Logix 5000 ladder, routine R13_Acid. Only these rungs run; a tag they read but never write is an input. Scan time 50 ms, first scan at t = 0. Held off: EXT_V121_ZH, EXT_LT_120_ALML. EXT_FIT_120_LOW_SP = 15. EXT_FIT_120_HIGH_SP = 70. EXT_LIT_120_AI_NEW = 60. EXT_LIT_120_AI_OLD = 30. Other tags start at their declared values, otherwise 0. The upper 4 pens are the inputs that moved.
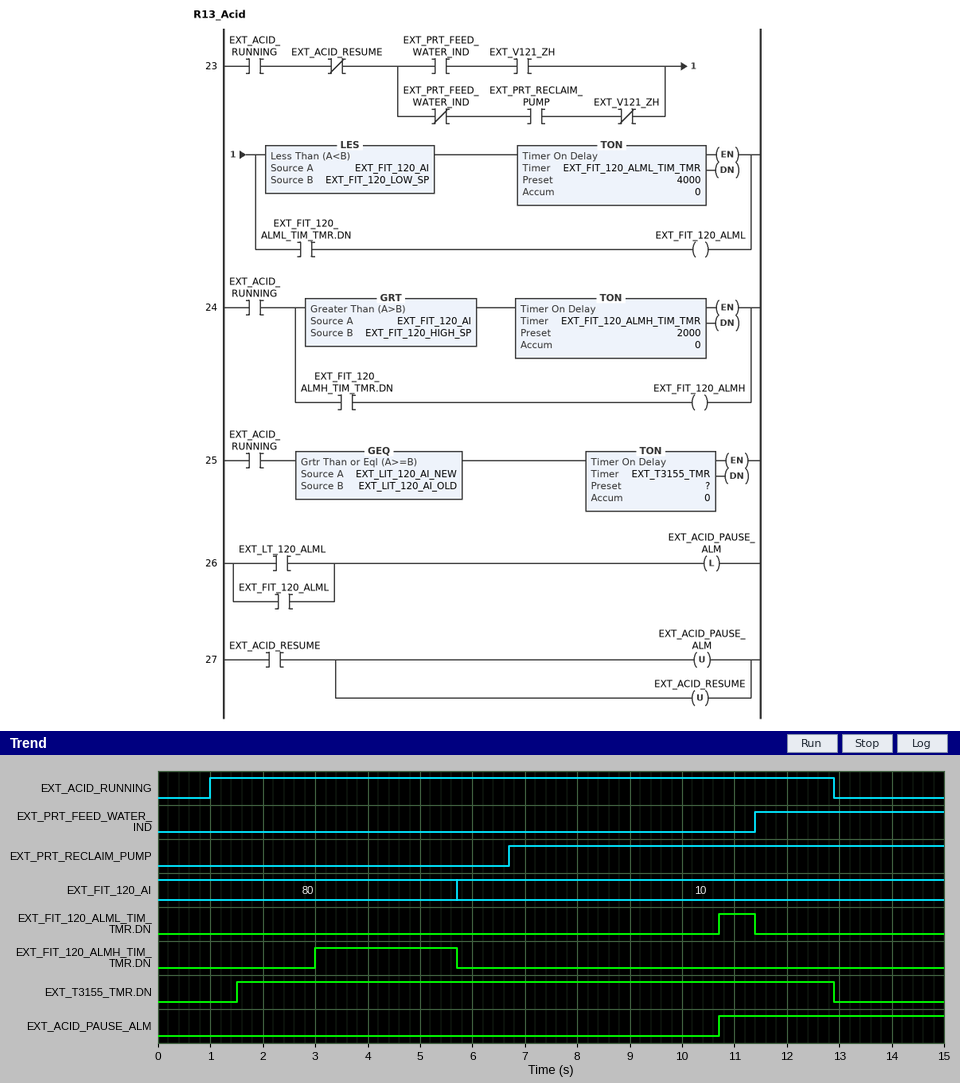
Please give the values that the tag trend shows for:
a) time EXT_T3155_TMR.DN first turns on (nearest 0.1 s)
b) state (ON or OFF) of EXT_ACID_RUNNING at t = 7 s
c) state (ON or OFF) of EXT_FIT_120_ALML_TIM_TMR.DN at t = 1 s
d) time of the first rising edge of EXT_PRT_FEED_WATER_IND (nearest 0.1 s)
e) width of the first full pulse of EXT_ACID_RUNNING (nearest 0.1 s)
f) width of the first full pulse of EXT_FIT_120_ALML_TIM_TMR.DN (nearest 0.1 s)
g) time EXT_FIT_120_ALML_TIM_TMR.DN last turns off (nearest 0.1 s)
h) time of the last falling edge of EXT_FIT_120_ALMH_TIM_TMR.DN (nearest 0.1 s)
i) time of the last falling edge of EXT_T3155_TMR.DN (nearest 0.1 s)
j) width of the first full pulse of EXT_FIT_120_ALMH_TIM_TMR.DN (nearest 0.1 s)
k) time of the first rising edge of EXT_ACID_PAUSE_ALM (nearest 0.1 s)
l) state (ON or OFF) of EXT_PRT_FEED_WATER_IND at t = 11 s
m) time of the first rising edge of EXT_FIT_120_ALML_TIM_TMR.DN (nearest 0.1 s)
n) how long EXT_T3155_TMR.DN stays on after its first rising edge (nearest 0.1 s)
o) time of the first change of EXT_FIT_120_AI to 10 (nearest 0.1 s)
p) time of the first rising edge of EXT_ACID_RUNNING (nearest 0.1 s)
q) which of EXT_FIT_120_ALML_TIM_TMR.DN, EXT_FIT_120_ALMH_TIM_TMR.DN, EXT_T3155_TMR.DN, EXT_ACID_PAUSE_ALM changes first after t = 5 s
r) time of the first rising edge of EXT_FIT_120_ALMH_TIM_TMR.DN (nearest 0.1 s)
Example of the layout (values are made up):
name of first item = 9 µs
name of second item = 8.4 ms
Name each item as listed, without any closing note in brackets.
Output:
time EXT_T3155_TMR.DN first turns on = 1.5 s
state (ON or OFF) of EXT_ACID_RUNNING at t = 7 s = ON
state (ON or OFF) of EXT_FIT_120_ALML_TIM_TMR.DN at t = 1 s = OFF
time of the first rising edge of EXT_PRT_FEED_WATER_IND = 11.4 s
width of the first full pulse of EXT_ACID_RUNNING = 11.9 s
width of the first full pulse of EXT_FIT_120_ALML_TIM_TMR.DN = 0.7 s
time EXT_FIT_120_ALML_TIM_TMR.DN last turns off = 11.4 s
time of the last falling edge of EXT_FIT_120_ALMH_TIM_TMR.DN = 5.7 s
time of the last falling edge of EXT_T3155_TMR.DN = 12.9 s
width of the first full pulse of EXT_FIT_120_ALMH_TIM_TMR.DN = 2.7 s
time of the first rising edge of EXT_ACID_PAUSE_ALM = 10.7 s
state (ON or OFF) of EXT_PRT_FEED_WATER_IND at t = 11 s = OFF
time of the first rising edge of EXT_FIT_120_ALML_TIM_TMR.DN = 10.7 s
how long EXT_T3155_TMR.DN stays on after its first rising edge = 11.4 s
time of the first change of EXT_FIT_120_AI to 10 = 5.7 s
time of the first rising edge of EXT_ACID_RUNNING = 1.0 s
which of EXT_FIT_120_ALML_TIM_TMR.DN, EXT_FIT_120_ALMH_TIM_TMR.DN, EXT_T3155_TMR.DN, EXT_ACID_PAUSE_ALM changes first after t = 5 s = EXT_FIT_120_ALMH_TIM_TMR.DN
time of the first rising edge of EXT_FIT_120_ALMH_TIM_TMR.DN = 3.0 s
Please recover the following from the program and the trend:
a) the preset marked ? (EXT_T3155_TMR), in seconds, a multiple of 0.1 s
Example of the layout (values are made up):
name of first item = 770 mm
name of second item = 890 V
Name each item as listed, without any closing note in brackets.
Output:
the preset marked ? (EXT_T3155_TMR), in seconds, a multiple of 0.1 s = 0.5 s
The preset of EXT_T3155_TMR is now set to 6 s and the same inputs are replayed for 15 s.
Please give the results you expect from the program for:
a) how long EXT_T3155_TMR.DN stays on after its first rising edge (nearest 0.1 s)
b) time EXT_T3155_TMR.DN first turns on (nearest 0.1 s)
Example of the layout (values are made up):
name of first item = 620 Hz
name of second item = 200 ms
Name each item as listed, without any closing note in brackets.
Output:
how long EXT_T3155_TMR.DN stays on after its first rising edge = 5.9 s
time EXT_T3155_TMR.DN first turns on = 7.0 s
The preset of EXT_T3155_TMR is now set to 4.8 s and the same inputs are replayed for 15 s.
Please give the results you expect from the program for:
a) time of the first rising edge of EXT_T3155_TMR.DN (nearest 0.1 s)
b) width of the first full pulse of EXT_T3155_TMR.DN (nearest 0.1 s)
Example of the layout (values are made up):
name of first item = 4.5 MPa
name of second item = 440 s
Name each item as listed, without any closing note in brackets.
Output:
time of the first rising edge of EXT_T3155_TMR.DN = 5.8 s
width of the first full pulse of EXT_T3155_TMR.DN = 7.1 s
